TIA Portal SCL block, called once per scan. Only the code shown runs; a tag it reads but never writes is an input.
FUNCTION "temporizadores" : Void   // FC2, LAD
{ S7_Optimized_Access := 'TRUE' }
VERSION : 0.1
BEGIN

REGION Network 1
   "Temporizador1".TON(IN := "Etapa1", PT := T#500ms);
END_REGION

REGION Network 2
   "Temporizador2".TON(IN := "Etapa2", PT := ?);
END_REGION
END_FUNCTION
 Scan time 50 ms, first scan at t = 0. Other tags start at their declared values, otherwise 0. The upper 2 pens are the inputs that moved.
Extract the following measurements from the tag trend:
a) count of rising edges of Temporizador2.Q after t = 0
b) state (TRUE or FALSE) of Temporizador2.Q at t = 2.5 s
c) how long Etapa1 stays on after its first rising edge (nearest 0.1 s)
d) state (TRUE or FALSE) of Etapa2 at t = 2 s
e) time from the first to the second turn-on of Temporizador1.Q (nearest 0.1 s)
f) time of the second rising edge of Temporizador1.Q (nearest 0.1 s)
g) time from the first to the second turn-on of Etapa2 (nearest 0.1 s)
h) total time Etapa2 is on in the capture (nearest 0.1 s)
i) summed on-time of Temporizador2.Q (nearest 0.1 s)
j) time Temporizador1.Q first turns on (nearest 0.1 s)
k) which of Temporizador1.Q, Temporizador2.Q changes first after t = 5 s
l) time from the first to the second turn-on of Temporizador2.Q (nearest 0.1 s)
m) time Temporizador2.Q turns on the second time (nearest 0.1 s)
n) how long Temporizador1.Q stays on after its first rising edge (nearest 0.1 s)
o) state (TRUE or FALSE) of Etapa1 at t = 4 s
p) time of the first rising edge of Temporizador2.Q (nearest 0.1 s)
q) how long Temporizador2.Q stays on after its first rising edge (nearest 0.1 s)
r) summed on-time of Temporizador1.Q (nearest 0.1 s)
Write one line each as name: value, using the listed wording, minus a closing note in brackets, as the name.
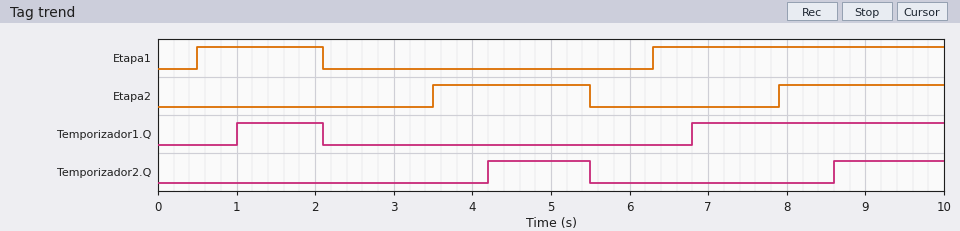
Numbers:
count of rising edges of Temporizador2.Q after t = 0: 2
state (TRUE or FALSE) of Temporizador2.Q at t = 2.5 s: FALSE
how long Etapa1 stays on after its first rising edge: 1.6 s
state (TRUE or FALSE) of Etapa2 at t = 2 s: FALSE
time from the first to the second turn-on of Temporizador1.Q: 5.8 s
time of the second rising edge of Temporizador1.Q: 6.8 s
time from the first to the second turn-on of Etapa2: 4.4 s
total time Etapa2 is on in the capture: 4.1 s
summed on-time of Temporizador2.Q: 2.7 s
time Temporizador1.Q first turns on: 1.0 s
which of Temporizador1.Q, Temporizador2.Q changes first after t = 5 s: Temporizador2.Q
time from the first to the second turn-on of Temporizador2.Q: 4.4 s
time Temporizador2.Q turns on the second time: 8.6 s
how long Temporizador1.Q stays on after its first rising edge: 1.1 s
state (TRUE or FALSE) of Etapa1 at t = 4 s: FALSE
time of the first rising edge of Temporizador2.Q: 4.2 s
how long Temporizador2.Q stays on after its first rising edge: 1.3 s
summed on-time of Temporizador1.Q: 4.3 s
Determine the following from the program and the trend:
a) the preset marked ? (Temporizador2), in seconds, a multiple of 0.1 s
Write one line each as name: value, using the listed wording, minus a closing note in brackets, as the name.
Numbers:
the preset marked ? (Temporizador2), in seconds, a multiple of 0.1 s: 0.7 s
